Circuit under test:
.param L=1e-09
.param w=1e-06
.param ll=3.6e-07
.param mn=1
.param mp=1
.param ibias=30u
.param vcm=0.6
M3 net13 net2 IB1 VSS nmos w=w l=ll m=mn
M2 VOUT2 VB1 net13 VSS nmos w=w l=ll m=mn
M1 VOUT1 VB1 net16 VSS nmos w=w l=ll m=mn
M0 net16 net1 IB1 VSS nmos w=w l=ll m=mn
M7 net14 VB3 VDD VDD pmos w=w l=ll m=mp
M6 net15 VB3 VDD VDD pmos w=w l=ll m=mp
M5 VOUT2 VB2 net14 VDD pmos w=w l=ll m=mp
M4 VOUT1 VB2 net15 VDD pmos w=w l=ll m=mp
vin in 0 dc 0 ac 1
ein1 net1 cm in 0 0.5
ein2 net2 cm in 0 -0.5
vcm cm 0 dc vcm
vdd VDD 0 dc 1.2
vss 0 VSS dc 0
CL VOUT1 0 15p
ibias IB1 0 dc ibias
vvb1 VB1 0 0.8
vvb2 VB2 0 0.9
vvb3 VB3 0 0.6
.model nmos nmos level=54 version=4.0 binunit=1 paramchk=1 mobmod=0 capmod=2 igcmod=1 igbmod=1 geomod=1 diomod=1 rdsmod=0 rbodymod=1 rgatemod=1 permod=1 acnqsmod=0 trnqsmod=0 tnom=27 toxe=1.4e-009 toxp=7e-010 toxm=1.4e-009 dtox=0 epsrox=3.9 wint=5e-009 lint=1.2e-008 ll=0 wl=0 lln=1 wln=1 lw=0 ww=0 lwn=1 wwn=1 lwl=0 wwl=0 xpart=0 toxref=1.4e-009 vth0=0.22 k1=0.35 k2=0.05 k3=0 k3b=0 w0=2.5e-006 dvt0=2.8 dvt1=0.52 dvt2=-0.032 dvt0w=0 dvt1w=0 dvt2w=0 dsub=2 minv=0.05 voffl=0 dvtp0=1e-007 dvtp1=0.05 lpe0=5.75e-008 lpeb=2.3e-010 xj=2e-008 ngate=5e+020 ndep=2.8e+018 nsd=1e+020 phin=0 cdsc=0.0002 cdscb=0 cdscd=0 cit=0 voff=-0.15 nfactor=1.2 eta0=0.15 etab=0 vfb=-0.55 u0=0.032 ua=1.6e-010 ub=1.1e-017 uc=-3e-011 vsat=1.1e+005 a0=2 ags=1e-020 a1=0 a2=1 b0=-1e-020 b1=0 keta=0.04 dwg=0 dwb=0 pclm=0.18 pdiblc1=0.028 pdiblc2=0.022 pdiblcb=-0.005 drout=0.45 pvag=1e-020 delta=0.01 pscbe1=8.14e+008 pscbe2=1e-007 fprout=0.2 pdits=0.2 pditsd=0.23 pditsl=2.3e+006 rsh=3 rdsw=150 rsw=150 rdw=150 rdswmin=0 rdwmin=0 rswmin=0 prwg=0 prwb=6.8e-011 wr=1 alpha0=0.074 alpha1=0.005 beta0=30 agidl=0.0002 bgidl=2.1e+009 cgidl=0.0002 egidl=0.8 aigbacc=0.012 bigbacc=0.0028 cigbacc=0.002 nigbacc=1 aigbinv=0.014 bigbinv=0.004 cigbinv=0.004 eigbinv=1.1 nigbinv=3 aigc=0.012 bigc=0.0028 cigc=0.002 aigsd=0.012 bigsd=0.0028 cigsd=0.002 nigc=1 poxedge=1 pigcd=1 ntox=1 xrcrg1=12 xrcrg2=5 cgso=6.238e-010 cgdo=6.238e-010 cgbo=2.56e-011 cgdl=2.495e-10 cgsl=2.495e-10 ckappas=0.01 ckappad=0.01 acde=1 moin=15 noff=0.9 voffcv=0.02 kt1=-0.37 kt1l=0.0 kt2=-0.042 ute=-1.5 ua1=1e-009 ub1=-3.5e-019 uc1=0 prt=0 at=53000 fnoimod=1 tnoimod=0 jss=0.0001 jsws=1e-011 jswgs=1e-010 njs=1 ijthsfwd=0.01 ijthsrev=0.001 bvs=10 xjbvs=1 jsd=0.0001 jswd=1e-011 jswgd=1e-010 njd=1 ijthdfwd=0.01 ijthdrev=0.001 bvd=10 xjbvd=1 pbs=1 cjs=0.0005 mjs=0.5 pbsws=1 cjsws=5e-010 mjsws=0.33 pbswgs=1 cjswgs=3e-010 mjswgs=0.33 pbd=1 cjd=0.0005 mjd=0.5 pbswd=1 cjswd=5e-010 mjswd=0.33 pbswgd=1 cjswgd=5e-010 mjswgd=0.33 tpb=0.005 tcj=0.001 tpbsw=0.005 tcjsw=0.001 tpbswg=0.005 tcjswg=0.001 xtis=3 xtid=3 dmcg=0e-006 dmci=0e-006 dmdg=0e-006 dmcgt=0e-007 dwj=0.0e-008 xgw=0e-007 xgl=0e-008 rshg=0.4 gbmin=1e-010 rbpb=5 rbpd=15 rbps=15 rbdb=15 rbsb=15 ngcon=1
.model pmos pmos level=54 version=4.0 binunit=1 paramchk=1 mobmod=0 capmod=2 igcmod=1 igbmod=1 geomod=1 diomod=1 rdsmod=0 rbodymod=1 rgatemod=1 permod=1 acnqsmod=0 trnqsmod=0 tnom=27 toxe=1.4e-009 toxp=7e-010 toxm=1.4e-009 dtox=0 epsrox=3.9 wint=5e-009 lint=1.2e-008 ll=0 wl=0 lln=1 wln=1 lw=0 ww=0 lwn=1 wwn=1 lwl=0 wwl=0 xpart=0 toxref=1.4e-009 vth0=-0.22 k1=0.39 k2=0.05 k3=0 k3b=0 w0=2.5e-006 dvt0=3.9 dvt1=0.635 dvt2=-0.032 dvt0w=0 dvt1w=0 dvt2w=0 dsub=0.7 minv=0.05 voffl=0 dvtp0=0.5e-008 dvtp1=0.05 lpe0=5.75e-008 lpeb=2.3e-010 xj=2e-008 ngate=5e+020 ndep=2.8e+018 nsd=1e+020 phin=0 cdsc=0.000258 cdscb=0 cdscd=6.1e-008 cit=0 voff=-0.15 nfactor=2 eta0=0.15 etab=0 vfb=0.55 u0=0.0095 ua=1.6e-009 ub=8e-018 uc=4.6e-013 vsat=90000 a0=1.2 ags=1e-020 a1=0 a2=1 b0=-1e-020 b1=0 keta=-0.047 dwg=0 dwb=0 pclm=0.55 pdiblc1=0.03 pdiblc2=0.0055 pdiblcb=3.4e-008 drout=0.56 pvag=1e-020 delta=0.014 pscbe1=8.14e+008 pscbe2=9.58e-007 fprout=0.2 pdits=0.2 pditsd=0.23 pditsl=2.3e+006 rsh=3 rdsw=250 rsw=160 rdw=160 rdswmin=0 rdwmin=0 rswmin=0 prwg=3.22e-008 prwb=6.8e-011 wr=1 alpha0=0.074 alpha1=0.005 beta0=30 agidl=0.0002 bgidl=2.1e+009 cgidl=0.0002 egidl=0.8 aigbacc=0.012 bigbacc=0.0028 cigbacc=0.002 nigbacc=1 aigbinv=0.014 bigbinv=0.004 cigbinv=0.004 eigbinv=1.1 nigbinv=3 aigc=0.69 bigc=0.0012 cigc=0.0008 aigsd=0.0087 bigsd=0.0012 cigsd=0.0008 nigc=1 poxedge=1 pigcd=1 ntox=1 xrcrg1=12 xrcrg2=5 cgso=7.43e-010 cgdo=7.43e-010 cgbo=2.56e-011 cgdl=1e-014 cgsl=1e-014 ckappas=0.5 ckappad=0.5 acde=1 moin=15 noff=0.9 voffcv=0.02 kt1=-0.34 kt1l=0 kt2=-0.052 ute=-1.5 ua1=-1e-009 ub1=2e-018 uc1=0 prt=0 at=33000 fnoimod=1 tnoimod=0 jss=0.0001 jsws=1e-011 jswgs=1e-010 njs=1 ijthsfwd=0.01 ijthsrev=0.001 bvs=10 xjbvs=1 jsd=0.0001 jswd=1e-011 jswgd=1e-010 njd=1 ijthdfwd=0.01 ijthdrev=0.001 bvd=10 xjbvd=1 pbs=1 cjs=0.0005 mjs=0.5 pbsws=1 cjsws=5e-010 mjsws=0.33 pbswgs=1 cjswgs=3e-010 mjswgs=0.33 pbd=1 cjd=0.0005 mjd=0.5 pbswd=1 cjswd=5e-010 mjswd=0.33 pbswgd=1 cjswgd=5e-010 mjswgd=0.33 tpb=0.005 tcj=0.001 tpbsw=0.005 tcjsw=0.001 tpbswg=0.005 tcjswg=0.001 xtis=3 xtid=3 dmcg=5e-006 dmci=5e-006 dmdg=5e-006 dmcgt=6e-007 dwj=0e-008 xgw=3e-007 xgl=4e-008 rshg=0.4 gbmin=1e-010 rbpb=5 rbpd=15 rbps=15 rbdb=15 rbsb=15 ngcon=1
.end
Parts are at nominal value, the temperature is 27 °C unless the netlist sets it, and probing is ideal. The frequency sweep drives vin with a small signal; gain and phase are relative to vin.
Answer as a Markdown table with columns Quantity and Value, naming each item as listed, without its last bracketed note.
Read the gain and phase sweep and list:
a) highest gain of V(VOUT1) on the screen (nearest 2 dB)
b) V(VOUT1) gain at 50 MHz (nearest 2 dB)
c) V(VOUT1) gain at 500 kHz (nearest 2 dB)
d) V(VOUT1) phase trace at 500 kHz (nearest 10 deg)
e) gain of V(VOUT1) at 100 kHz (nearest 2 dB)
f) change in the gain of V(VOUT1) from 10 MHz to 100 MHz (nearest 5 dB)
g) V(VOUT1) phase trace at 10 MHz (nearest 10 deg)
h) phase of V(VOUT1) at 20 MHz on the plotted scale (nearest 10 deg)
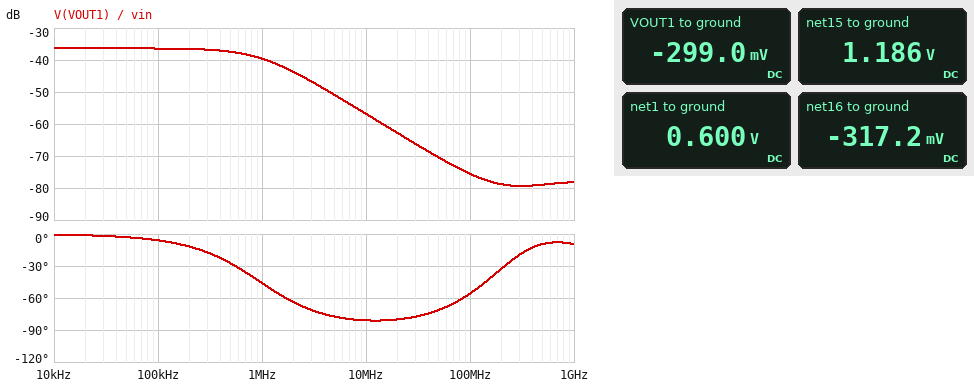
| Quantity | Value |
|---|---|
| highest gain of V(VOUT1) on the screen | -36 dB |
| V(VOUT1) gain at 50 MHz | -70 dB |
| V(VOUT1) gain at 500 kHz | -38 dB |
| V(VOUT1) phase trace at 500 kHz | -30 deg |
| gain of V(VOUT1) at 100 kHz | -36 dB |
| change in the gain of V(VOUT1) from 10 MHz to 100 MHz | -20 dB |
| V(VOUT1) phase trace at 10 MHz | -80 deg |
| phase of V(VOUT1) at 20 MHz on the plotted scale | -80 deg |
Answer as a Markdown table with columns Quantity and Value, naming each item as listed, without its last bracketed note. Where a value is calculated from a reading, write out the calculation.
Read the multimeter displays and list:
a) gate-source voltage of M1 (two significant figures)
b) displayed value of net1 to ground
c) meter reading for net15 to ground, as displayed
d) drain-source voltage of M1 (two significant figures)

| Quantity | Value |
|---|---|
| gate-source voltage of M1 | 800 mV - (-317.2 mV) = 1.1 V |
| displayed value of net1 to ground | 0.600 V |
| meter reading for net15 to ground, as displayed | 1.186 V |
| drain-source voltage of M1 | -299 mV - (-317.2 mV) = 18 mV |
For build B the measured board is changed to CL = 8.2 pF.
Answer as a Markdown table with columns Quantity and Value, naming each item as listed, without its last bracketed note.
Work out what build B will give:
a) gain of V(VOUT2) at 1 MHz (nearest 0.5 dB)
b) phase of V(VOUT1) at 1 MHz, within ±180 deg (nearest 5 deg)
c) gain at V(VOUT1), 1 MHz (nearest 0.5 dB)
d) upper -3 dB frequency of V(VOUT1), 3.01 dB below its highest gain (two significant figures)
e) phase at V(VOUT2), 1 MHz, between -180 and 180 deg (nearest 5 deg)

| Quantity | Value |
|---|---|
| gain of V(VOUT2) at 1 MHz | -35.0 dB |
| phase of V(VOUT1) at 1 MHz, within ±180 deg | -30 deg |
| gain at V(VOUT1), 1 MHz | -37.5 dB |
| upper -3 dB frequency of V(VOUT1), 3.01 dB below its highest gain | 1.7 MHz |
| phase at V(VOUT2), 1 MHz, between -180 and 180 deg | -170 deg |
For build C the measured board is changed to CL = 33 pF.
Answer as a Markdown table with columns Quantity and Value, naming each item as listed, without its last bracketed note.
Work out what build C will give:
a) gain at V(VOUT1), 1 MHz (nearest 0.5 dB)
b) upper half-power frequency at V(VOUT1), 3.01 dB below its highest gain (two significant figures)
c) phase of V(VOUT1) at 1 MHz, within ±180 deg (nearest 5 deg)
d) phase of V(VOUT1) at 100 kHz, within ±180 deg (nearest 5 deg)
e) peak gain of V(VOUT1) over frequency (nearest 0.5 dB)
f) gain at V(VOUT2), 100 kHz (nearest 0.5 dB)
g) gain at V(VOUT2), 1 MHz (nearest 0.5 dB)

| Quantity | Value |
|---|---|
| gain at V(VOUT1), 1 MHz | -44.5 dB |
| upper half-power frequency at V(VOUT1), 3.01 dB below its highest gain | 430 kHz |
| phase of V(VOUT1) at 1 MHz, within ±180 deg | -65 deg |
| phase of V(VOUT1) at 100 kHz, within ±180 deg | -15 deg |
| peak gain of V(VOUT1) over frequency | -36.5 dB |
| gain at V(VOUT2), 100 kHz | -36.0 dB |
| gain at V(VOUT2), 1 MHz | -33.5 dB |
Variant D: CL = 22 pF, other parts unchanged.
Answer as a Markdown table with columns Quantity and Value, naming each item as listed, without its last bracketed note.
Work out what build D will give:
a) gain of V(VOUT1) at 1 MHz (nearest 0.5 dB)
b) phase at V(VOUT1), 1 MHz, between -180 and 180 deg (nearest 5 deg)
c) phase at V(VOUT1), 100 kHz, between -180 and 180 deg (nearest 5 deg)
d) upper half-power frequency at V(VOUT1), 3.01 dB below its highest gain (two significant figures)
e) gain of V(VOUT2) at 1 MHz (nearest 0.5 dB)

| Quantity | Value |
|---|---|
| gain of V(VOUT1) at 1 MHz | -41.5 dB |
| phase at V(VOUT1), 1 MHz, between -180 and 180 deg | -55 deg |
| phase at V(VOUT1), 100 kHz, between -180 and 180 deg | -10 deg |
| upper half-power frequency at V(VOUT1), 3.01 dB below its highest gain | 650 kHz |
| gain of V(VOUT2) at 1 MHz | -33.5 dB |
